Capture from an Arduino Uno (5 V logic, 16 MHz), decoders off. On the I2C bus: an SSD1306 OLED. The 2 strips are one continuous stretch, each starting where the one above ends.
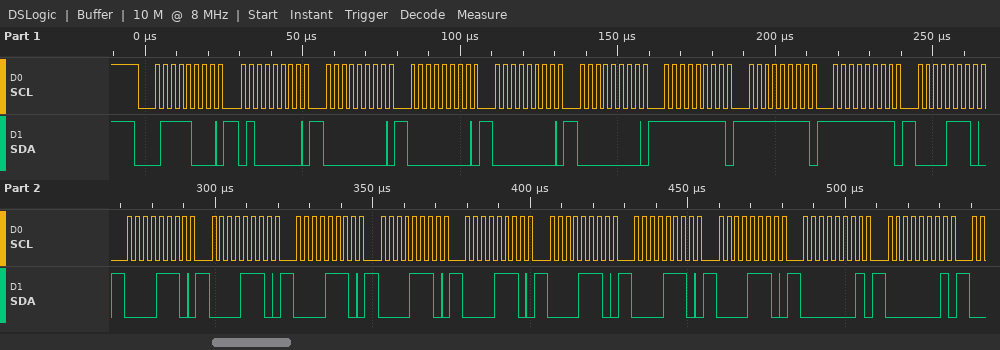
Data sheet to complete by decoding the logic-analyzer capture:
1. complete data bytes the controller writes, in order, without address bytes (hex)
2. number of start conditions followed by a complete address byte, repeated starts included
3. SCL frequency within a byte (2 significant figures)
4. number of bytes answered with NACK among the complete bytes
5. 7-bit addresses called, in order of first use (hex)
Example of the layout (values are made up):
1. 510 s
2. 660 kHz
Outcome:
1. 40 00 00 00 00 FF FF FF 0E 0E 0E 0E 0E 0E 0E 0E 0E 01 01
2. 1
3. 400 kHz
4. 0
5. 0x3C
